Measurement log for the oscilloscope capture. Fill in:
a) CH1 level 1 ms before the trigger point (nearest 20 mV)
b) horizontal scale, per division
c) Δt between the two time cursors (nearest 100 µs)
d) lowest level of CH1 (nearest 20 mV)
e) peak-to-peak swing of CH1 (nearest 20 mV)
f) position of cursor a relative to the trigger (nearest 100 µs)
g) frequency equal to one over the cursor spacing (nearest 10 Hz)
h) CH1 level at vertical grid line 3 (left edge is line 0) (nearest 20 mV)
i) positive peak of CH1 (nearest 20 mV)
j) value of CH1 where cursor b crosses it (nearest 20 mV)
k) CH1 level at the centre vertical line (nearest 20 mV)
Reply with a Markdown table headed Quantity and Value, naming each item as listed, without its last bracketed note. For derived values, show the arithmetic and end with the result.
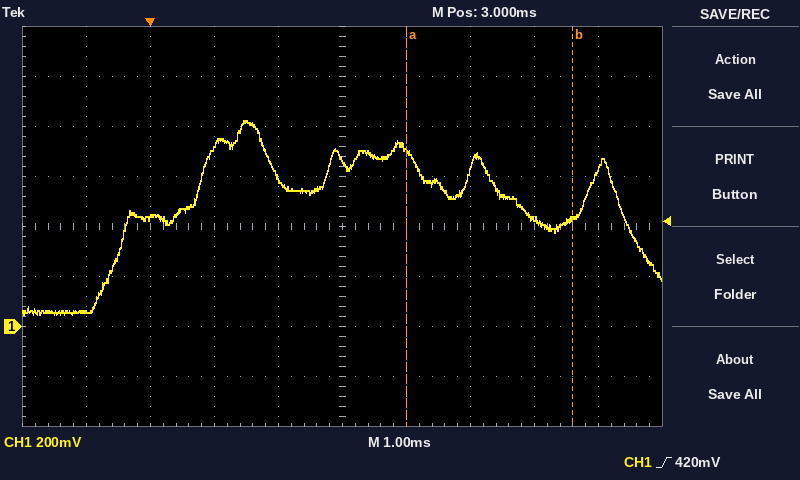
| Quantity | Value |
|---|---|
| CH1 level 1 ms before the trigger point | 60 mV |
| horizontal scale, per division | 1 ms |
| Δt between the two time cursors | 2.6 ms |
| lowest level of CH1 | 40 mV |
| peak-to-peak swing of CH1 | 820 mV − (40 mV) = 780 mV |
| position of cursor a relative to the trigger | +4.0 ms |
| frequency equal to one over the cursor spacing | 1 / 2.6 ms ≈ 380 Hz |
| CH1 level at vertical grid line 3 (left edge is line 0) | 720 mV |
| positive peak of CH1 | 820 mV |
| value of CH1 where cursor b crosses it | 420 mV |
| CH1 level at the centre vertical line | 660 mV |
